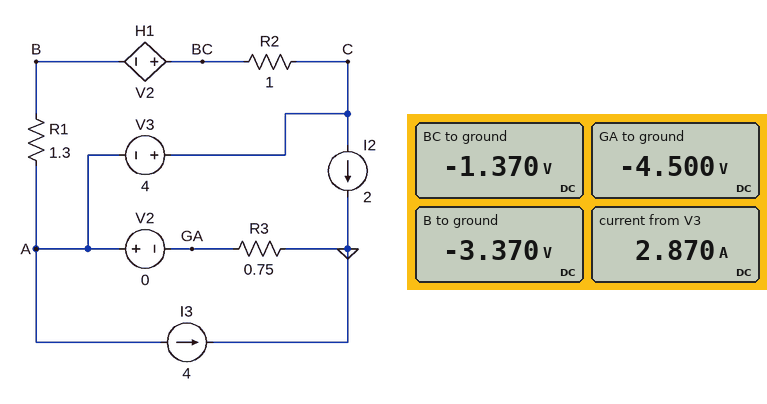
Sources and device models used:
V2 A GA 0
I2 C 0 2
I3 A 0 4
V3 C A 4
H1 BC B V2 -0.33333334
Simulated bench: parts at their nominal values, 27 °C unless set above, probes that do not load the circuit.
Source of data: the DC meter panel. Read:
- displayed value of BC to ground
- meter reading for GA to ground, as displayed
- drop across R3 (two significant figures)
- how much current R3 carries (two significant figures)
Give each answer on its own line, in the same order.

-1.370 V
-4.500 V
4.5 V
6.0 A
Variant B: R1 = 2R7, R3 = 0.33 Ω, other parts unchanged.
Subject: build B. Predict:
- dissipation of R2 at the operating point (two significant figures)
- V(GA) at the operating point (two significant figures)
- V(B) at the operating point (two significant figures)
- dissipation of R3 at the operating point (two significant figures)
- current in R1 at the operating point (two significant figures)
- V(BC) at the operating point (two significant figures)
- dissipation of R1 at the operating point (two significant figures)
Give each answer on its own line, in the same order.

290 mW
-2.0 V
-520 mV
12 W
540 mA
1.5 V
790 mW
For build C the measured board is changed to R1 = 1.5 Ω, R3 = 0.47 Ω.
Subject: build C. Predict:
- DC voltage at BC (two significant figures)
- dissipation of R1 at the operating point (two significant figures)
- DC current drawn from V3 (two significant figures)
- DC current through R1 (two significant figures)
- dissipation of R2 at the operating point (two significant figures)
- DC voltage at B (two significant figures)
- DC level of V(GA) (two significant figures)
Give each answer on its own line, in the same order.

380 mV
960 mW
2.8 A
800 mA
640 mW
-1.6 V
-2.8 V
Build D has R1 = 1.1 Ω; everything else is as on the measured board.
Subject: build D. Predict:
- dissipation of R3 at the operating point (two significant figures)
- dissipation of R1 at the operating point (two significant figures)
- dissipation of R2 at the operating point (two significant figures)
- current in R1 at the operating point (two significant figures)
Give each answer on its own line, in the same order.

27 W
1.0 W
910 mW
950 mA
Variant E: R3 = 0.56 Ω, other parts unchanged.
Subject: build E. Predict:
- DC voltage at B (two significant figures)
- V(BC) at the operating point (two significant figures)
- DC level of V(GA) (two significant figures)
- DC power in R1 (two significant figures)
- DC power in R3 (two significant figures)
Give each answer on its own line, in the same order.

-2.2 V
-230 mV
-3.4 V
980 mW
20 W
